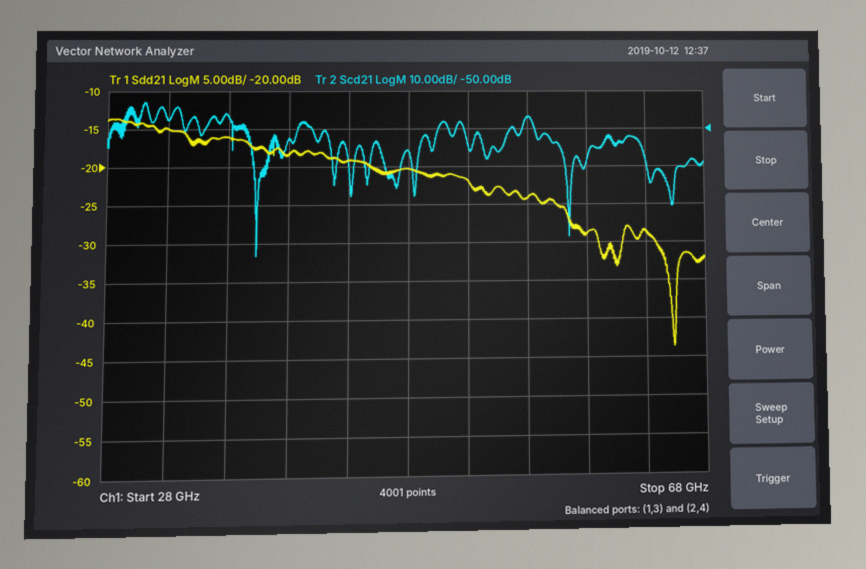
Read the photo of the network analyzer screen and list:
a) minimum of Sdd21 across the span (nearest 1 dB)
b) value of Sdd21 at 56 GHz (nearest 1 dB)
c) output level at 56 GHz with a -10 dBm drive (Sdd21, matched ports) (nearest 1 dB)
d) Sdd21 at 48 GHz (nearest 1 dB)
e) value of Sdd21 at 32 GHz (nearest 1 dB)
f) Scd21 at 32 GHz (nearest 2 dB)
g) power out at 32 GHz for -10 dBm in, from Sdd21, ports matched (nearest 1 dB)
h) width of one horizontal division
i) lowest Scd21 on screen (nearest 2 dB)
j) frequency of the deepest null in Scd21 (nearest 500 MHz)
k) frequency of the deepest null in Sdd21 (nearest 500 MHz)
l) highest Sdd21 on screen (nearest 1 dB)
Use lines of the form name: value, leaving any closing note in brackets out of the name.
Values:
minimum of Sdd21 across the span: -44 dB
value of Sdd21 at 56 GHz: -24 dB
output level at 56 GHz with a -10 dBm drive (Sdd21, matched ports): -34 dBm
Sdd21 at 48 GHz: -20 dB
value of Sdd21 at 32 GHz: -15 dB
Scd21 at 32 GHz: -48 dB
power out at 32 GHz for -10 dBm in, from Sdd21, ports matched: -25 dBm
width of one horizontal division: 4 GHz
lowest Scd21 on screen: -84 dB
frequency of the deepest null in Scd21: 38.0 GHz
frequency of the deepest null in Sdd21: 66.0 GHz
highest Sdd21 on screen: -14 dB
